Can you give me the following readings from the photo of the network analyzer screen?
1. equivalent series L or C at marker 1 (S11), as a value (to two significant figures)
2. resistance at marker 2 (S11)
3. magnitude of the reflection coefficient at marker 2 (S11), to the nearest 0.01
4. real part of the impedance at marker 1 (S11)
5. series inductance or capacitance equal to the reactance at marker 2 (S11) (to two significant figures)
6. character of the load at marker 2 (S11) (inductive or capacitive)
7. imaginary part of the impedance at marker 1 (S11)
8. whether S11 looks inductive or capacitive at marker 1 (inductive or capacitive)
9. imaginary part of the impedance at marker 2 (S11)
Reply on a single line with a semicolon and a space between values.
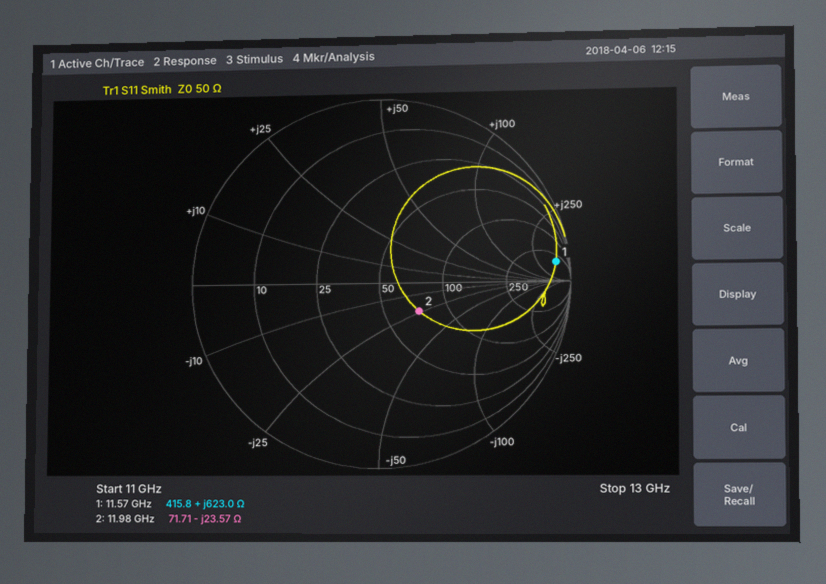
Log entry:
8.6 nH; 71.71 Ω; 0.26; 415.8 Ω; 560 fF; capacitive; +623.0 Ω; inductive; -23.57 Ω
